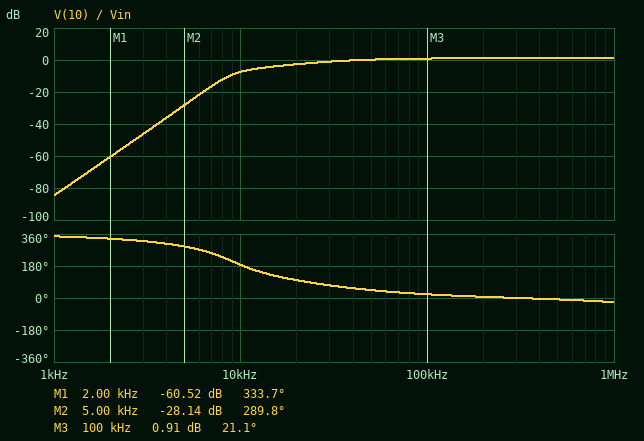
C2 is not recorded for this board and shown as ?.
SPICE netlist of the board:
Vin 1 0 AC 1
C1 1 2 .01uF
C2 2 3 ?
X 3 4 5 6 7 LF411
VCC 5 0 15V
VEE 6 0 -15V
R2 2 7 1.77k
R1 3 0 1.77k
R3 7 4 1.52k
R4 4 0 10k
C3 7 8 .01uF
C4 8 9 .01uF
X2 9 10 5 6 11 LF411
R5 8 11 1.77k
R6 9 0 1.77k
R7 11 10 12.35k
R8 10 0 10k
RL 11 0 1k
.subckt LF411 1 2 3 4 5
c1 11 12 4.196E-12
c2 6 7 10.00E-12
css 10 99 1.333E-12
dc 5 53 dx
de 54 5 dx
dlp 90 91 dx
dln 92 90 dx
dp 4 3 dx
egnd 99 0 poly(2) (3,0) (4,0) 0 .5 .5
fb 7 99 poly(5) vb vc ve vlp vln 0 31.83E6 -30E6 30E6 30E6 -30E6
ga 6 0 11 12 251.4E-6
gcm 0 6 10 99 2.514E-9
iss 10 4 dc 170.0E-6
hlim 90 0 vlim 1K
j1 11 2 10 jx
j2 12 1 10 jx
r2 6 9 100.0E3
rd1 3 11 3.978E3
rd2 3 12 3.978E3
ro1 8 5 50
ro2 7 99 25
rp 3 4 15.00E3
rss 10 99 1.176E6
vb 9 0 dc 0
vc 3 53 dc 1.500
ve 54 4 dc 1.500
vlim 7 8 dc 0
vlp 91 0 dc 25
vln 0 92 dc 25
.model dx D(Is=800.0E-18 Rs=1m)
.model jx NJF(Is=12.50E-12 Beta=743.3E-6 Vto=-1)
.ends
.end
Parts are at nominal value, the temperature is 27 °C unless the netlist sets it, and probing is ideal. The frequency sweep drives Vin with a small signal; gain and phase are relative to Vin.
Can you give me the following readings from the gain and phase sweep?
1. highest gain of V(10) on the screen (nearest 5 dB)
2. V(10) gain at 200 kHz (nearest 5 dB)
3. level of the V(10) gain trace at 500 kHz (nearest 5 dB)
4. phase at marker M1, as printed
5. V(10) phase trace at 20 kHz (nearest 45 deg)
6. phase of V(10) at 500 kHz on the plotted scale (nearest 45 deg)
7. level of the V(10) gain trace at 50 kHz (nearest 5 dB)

0 dB
0 dB
0 dB
333.7 deg
90 deg
0 deg
0 dB
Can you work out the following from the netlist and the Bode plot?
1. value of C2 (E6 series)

3.3 nF
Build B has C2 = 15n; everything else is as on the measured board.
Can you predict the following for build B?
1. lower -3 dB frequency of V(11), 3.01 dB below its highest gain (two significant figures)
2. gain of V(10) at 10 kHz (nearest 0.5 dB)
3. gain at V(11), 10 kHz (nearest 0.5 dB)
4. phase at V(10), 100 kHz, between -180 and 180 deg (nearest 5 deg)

9.0 kHz
1.0 dB
8.0 dB
10 deg
